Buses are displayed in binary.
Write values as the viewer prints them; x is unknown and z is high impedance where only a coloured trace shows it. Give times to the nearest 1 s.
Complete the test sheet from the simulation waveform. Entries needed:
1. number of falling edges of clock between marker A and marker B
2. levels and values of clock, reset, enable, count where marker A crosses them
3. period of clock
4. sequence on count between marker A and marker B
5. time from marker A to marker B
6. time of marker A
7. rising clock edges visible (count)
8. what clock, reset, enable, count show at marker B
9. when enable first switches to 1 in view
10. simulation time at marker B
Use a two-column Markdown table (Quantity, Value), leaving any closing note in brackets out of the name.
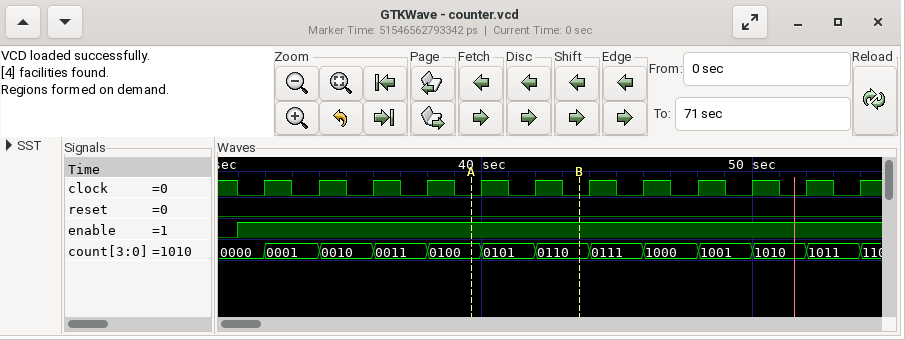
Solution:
| Quantity | Value |
|---|---|
| number of falling edges of clock between marker A and marker B | 2 |
| levels and values of clock, reset, enable, count where marker A crosses them | clock=0, reset=0, enable=1, count=0100 |
| period of clock | 2 s |
| sequence on count between marker A and marker B | 0100, 0101, 0110 |
| time from marker A to marker B | 4 s |
| time of marker A | 40 s |
| rising clock edges visible | 12 |
| what clock, reset, enable, count show at marker B | clock=0, reset=0, enable=1, count=0110 |
| when enable first switches to 1 in view | 31 s |
| simulation time at marker B | 44 s |
